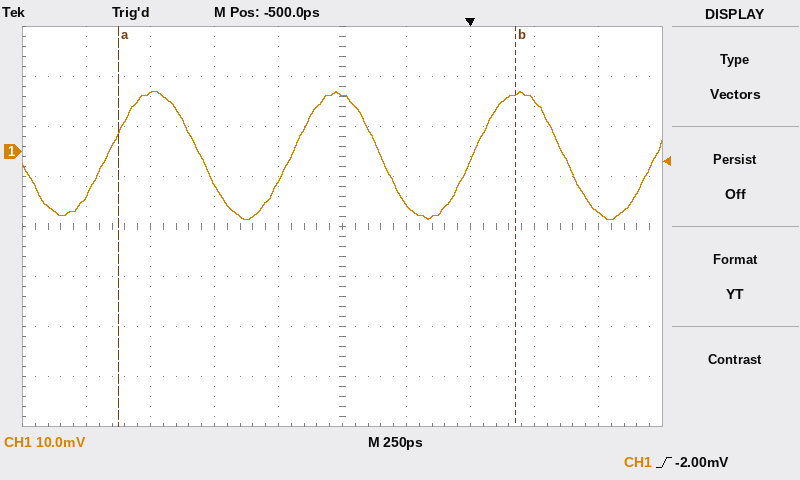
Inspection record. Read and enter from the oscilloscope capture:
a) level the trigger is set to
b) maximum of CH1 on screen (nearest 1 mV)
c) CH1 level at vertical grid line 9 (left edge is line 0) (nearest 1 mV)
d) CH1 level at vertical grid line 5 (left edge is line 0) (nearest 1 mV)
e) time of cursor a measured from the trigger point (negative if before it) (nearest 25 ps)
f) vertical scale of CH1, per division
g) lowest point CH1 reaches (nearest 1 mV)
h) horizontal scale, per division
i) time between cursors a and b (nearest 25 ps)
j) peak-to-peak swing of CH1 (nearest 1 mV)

-2.00 mV
12 mV
-12 mV
11 mV
-1.375 ns
10 mV
-14 mV
250 ps
1.550 ns
26 mV
